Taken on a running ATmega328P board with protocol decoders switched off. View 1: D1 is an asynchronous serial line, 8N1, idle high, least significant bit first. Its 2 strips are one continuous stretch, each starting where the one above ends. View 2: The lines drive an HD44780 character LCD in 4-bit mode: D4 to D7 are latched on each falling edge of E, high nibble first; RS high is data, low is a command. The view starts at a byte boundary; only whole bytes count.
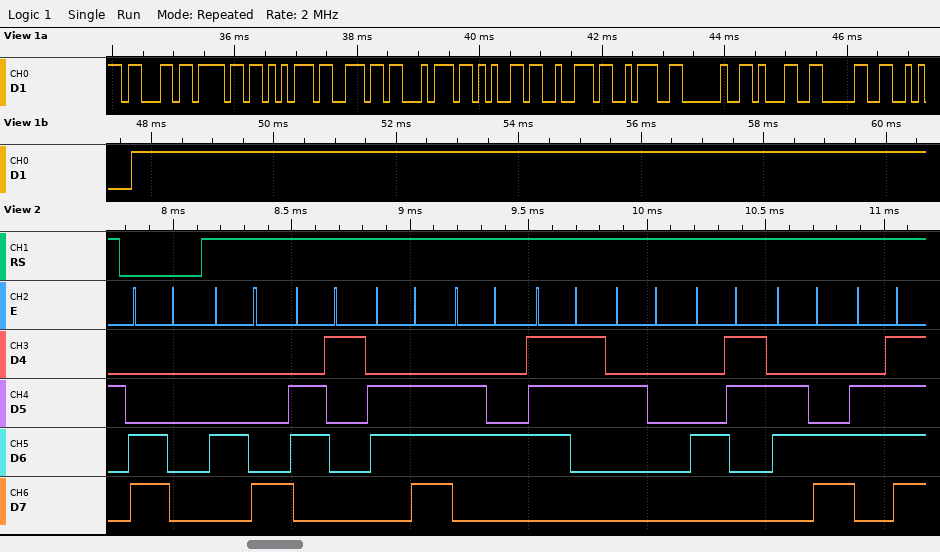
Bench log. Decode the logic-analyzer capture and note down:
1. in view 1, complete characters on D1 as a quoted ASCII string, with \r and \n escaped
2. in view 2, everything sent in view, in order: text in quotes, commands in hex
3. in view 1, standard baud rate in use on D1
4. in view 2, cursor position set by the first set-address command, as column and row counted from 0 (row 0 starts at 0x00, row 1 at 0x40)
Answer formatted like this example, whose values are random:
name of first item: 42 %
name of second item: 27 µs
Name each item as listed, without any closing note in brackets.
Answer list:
in view 1, complete characters on D1 as a quoted ASCII string, with \r and \n escaped: "counter: 10\n"
in view 2, everything sent in view, in order: text in quotes, commands in hex: 0xC0 "Hands Clo"
in view 1, standard baud rate in use on D1: 9600 baud
in view 2, cursor position set by the first set-address command, as column and row counted from 0: column 0, row 1
